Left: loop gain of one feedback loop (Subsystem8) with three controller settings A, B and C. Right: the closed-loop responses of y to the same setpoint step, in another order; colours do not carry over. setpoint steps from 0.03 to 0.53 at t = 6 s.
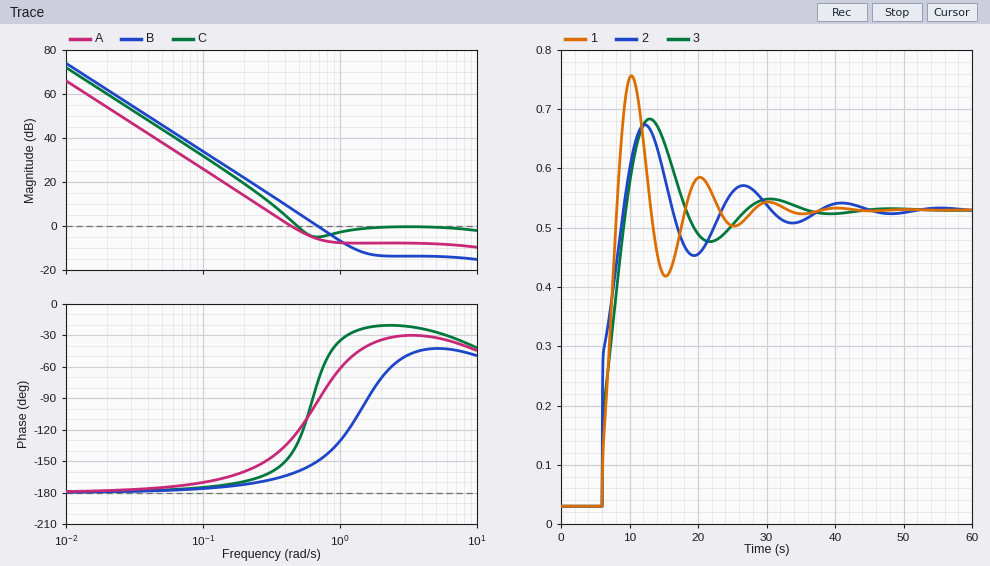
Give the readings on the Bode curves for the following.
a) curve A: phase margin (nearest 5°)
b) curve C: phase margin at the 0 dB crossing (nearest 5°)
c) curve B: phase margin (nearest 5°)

50°
45°
30°
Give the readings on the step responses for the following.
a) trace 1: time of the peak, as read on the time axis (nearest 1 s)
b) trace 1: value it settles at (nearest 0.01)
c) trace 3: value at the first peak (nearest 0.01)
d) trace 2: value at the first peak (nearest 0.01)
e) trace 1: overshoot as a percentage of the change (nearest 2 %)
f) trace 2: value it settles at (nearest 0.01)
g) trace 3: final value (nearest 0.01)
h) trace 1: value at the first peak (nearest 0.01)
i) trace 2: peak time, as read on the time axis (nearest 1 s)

10 s
0.53
0.68
0.67
46 %
0.53
0.53
0.76
12 s
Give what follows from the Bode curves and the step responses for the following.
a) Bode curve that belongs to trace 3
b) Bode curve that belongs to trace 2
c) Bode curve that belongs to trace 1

A
C
B
